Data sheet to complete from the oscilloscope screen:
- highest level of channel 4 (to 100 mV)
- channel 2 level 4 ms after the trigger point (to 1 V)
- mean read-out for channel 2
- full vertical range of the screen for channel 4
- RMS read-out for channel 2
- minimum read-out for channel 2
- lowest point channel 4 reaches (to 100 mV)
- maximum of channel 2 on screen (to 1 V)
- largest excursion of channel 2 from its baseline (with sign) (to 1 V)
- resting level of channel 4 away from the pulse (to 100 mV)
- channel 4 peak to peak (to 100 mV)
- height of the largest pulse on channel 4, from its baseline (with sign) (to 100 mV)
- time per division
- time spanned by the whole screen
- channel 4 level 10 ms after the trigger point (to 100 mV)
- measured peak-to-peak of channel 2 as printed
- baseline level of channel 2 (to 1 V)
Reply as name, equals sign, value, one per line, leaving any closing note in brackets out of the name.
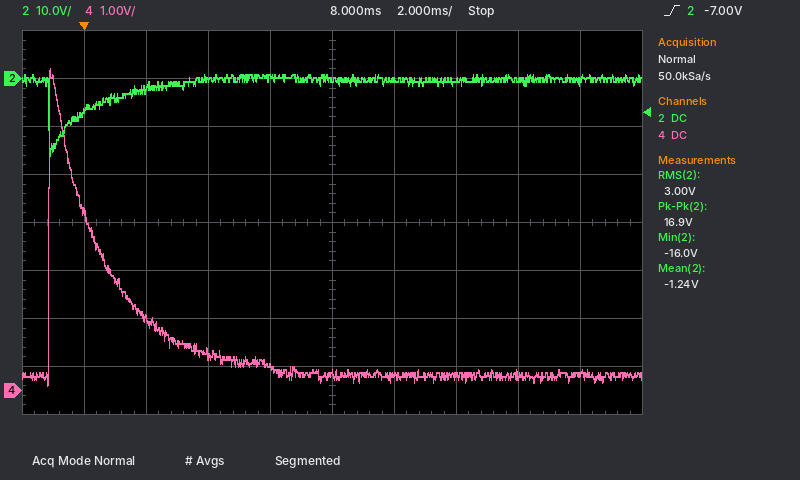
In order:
highest level of channel 4 = 6.7 V
channel 2 level 4 ms after the trigger point = 0 V
mean read-out for channel 2 = -1.24 V
full vertical range of the screen for channel 4 = 8 V
RMS read-out for channel 2 = 3.00 V
minimum read-out for channel 2 = -16.0 V
lowest point channel 4 reaches = 100 mV
maximum of channel 2 on screen = 1 V
largest excursion of channel 2 from its baseline (with sign) = -16 V
resting level of channel 4 away from the pulse = 300 mV
channel 4 peak to peak = 6.6 V
height of the largest pulse on channel 4, from its baseline (with sign) = +6.4 V
time per division = 2 ms
time spanned by the whole screen = 20 ms
channel 4 level 10 ms after the trigger point = 300 mV
measured peak-to-peak of channel 2 as printed = 16.9 V
baseline level of channel 2 = 0 V
